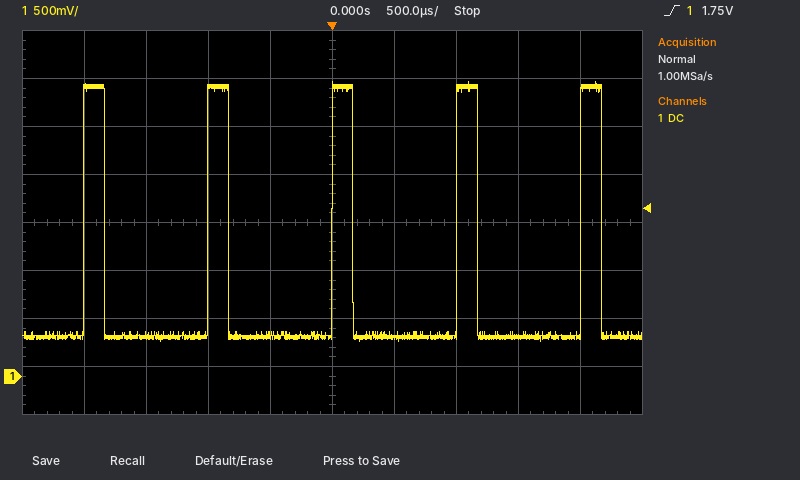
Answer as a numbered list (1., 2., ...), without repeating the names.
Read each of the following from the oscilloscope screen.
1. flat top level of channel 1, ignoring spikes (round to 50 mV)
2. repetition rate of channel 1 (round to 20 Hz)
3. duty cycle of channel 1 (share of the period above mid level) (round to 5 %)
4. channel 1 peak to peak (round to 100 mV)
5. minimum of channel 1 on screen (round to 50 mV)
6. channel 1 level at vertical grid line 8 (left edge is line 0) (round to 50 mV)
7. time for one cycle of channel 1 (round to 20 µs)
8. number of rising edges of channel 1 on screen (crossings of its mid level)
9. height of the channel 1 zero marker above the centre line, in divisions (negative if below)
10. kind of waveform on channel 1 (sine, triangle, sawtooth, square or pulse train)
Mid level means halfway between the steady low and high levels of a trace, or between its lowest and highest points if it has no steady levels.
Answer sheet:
1. 3.00 V
2. 1.00 kHz
3. 15 %
4. 2.70 V
5. 350 mV
6. 400 mV
7. 1.00 ms
8. 5
9. -3.2 div
10. pulse train
